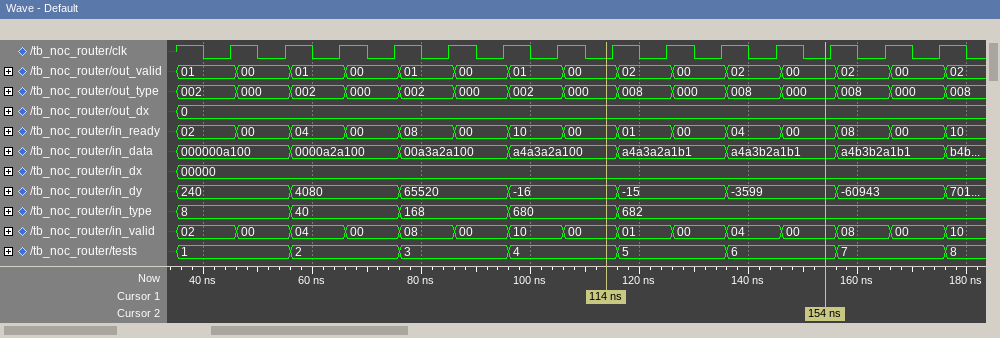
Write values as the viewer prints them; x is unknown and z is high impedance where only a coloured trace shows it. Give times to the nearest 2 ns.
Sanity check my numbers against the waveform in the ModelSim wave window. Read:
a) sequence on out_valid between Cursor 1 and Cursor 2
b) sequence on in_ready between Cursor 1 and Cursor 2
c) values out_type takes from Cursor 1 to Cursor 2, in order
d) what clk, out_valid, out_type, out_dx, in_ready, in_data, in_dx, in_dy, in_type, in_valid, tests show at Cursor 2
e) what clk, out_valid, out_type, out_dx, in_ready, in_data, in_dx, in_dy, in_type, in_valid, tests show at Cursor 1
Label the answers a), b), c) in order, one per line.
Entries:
a) 00, 02, 00, 02, 00
b) 00, 01, 00, 04, 00
c) 000, 008, 000, 008, 000
d) clk=0, out_valid=00, out_type=000, out_dx=0, in_ready=00, in_data=a4a3b2a1b1, in_dx=00000, in_dy=-3599, in_type=682, in_valid=00, tests=6
e) clk=0, out_valid=00, out_type=000, out_dx=0, in_ready=00, in_data=a4a3a2a100, in_dx=00000, in_dy=-16, in_type=680, in_valid=00, tests=4
